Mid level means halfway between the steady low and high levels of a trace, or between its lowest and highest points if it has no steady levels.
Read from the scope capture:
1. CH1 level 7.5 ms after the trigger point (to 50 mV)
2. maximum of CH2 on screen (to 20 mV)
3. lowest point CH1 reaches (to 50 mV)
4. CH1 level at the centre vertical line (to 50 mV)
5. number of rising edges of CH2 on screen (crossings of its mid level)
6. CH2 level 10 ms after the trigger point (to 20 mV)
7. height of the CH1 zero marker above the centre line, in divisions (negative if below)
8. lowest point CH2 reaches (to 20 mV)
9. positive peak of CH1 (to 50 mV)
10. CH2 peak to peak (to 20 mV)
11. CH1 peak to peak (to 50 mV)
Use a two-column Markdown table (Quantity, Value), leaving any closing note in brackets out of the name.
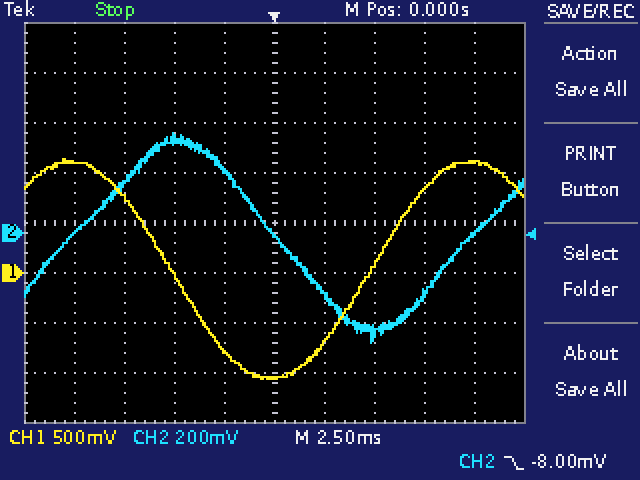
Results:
| Quantity | Value |
|---|---|
| CH1 level 7.5 ms after the trigger point | 850 mV |
| maximum of CH2 on screen | 400 mV |
| lowest point CH1 reaches | -1.05 V |
| CH1 level at the centre vertical line | -1.05 V |
| number of rising edges of CH2 on screen | 2 |
| CH2 level 10 ms after the trigger point | 0 mV |
| height of the CH1 zero marker above the centre line, in divisions | -1.0 div |
| lowest point CH2 reaches | -440 mV |
| positive peak of CH1 | 1.15 V |
| CH2 peak to peak | 840 mV |
| CH1 peak to peak | 2.20 V |
